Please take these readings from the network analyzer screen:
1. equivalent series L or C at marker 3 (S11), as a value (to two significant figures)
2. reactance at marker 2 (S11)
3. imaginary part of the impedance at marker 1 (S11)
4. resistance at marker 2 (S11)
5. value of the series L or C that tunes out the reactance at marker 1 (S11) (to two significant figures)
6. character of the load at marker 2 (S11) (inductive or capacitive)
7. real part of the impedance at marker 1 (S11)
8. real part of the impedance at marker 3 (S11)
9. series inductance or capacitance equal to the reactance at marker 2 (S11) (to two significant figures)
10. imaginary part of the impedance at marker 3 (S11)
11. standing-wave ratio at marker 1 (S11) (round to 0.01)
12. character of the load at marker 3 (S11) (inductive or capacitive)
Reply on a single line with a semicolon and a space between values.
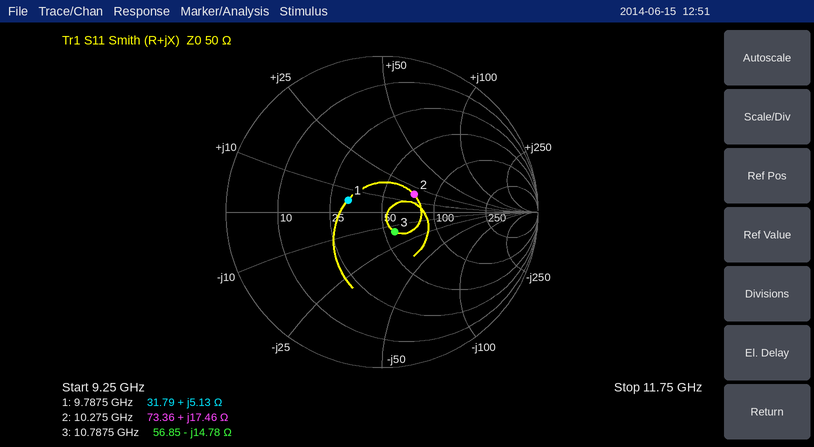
1.00 pF; +17.46 Ω; +5.13 Ω; 73.36 Ω; 3.2 pF; inductive; 31.79 Ω; 56.85 Ω; 270 pH; -14.78 Ω; 1.60; capacitive
